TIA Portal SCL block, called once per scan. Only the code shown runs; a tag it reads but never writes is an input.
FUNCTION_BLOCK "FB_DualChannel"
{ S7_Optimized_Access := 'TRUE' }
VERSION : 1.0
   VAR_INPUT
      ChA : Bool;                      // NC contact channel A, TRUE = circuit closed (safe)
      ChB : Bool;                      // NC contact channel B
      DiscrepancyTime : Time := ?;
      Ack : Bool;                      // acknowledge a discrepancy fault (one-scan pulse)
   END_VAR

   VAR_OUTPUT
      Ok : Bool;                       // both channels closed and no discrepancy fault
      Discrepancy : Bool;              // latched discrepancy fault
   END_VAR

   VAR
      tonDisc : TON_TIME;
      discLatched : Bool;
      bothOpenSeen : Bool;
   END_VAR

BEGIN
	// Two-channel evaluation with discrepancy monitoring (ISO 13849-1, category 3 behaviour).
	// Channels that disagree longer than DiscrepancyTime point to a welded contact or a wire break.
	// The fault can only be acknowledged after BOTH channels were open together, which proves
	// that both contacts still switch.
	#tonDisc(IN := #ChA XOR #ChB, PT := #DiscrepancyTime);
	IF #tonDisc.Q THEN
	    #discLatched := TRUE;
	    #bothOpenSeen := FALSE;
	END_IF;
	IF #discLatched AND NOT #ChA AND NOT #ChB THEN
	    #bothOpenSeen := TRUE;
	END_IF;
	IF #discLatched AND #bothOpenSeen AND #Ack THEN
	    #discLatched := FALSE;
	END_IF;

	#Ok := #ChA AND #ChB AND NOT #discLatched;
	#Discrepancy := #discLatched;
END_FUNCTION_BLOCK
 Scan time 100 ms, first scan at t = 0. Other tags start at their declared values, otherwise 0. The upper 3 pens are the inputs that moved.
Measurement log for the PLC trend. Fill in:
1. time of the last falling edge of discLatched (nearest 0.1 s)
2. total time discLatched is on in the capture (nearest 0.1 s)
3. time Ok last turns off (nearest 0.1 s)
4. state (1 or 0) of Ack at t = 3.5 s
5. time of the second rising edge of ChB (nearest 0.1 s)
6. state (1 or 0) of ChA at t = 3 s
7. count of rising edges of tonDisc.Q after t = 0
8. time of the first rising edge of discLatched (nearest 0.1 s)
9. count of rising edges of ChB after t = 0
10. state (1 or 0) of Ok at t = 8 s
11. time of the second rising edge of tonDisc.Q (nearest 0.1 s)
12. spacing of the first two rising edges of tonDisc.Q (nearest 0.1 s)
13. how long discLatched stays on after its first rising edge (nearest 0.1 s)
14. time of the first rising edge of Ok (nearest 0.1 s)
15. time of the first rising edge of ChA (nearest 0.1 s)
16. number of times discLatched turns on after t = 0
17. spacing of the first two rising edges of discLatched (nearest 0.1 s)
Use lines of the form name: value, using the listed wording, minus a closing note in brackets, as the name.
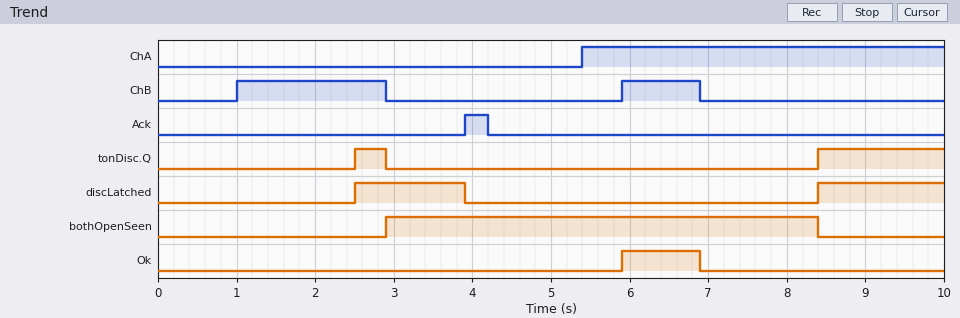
time of the last falling edge of discLatched: 3.9 s
total time discLatched is on in the capture: 3.0 s
time Ok last turns off: 6.9 s
state (1 or 0) of Ack at t = 3.5 s: 0
time of the second rising edge of ChB: 5.9 s
state (1 or 0) of ChA at t = 3 s: 0
count of rising edges of tonDisc.Q after t = 0: 2
time of the first rising edge of discLatched: 2.5 s
count of rising edges of ChB after t = 0: 2
state (1 or 0) of Ok at t = 8 s: 0
time of the second rising edge of tonDisc.Q: 8.4 s
spacing of the first two rising edges of tonDisc.Q: 5.9 s
how long discLatched stays on after its first rising edge: 1.4 s
time of the first rising edge of Ok: 5.9 s
time of the first rising edge of ChA: 5.4 s
number of times discLatched turns on after t = 0: 2
spacing of the first two rising edges of discLatched: 5.9 s
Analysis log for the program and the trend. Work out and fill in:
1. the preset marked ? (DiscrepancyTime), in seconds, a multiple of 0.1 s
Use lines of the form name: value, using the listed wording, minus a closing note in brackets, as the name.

the preset marked ? (DiscrepancyTime), in seconds, a multiple of 0.1 s: 1.5 s
